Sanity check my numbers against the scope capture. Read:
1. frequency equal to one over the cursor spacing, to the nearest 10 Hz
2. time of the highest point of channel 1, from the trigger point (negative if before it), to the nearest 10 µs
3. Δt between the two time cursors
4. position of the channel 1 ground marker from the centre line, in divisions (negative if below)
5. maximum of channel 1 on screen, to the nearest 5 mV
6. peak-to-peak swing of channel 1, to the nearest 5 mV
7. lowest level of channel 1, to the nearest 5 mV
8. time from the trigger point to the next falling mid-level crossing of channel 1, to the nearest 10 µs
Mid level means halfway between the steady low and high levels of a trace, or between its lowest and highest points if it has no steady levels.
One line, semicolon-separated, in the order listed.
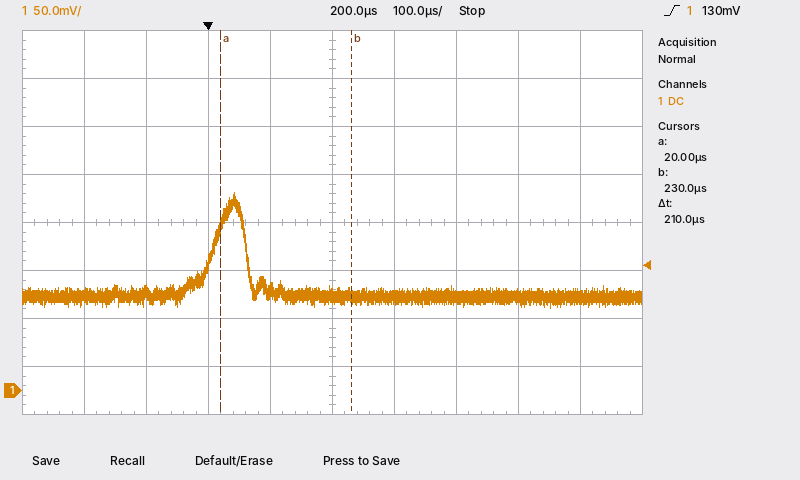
4.76 kHz; +40 µs; 210 µs; -3.5 div; 205 mV; 120 mV; 85 mV; 60 µs
